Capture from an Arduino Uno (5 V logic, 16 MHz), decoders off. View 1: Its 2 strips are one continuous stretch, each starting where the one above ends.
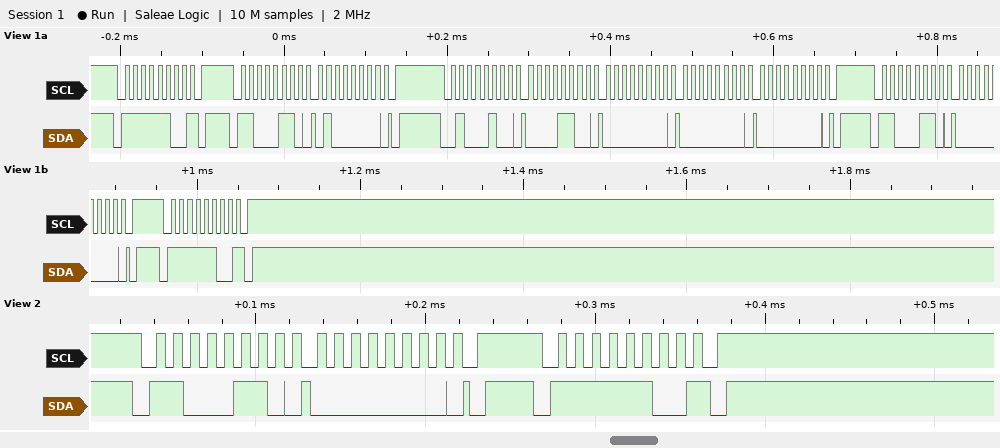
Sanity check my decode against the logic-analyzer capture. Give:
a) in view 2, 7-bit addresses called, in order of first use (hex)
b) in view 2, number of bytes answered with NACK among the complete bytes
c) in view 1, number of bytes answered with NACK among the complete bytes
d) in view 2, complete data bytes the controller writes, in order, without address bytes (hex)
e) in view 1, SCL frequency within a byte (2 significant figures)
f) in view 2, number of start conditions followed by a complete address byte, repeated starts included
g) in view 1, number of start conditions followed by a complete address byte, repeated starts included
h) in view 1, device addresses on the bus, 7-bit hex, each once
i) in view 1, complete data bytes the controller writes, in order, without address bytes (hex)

0x63 0x7E
1
2
00
100 kHz
2
5
0x7E 0x63 0x22
40 0C 00 00 00 00
